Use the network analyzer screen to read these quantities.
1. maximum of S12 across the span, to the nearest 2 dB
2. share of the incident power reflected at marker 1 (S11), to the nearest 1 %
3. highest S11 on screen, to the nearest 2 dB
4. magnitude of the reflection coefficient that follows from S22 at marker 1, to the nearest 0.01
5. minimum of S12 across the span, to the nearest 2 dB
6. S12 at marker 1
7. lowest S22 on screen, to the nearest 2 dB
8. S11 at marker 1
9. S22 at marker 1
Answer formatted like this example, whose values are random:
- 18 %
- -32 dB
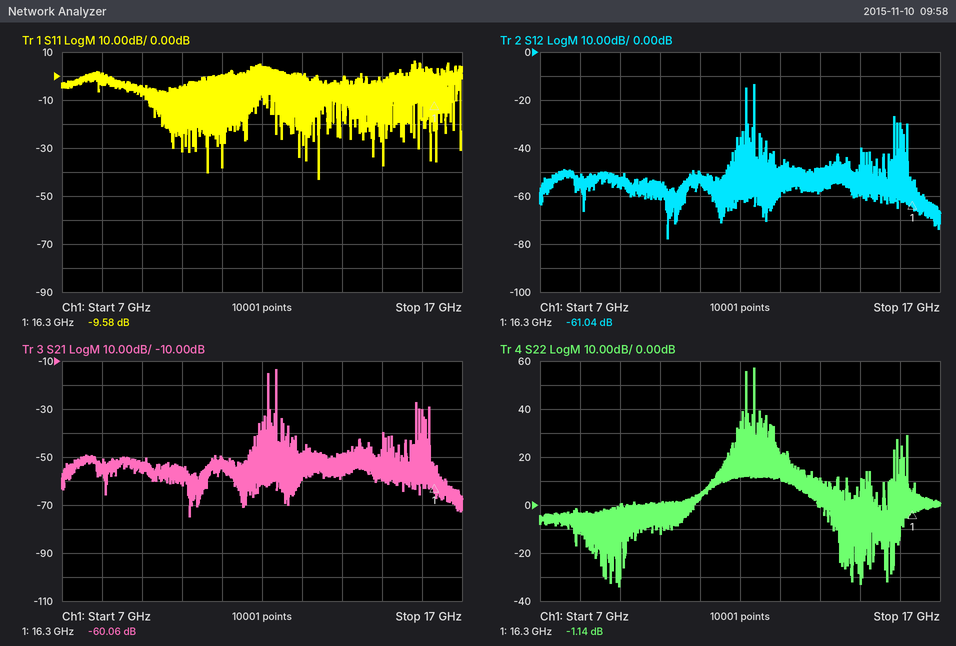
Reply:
- -14 dB
- 11 %
- 6 dB
- 0.88
- -78 dB
- -61.04 dB
- -34 dB
- -9.58 dB
- -1.14 dB
